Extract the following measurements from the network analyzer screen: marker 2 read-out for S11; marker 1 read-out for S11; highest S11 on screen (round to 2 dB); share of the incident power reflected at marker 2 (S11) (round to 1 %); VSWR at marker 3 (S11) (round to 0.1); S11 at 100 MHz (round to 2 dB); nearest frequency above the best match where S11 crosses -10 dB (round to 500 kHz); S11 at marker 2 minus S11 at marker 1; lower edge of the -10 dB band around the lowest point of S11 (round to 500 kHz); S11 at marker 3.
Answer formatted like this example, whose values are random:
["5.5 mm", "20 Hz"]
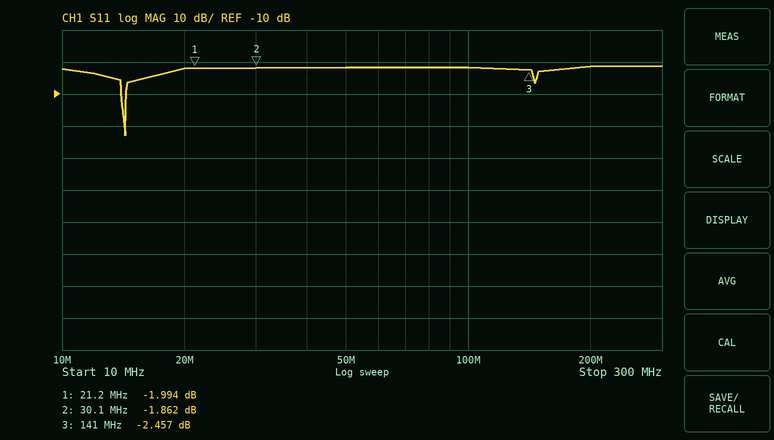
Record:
["-1.862 dB", "-1.994 dB", "-2 dB", "65 %", "7.1", "-2 dB", "14.5 MHz", "0.132 dB", "14.0 MHz", "-2.457 dB"]
